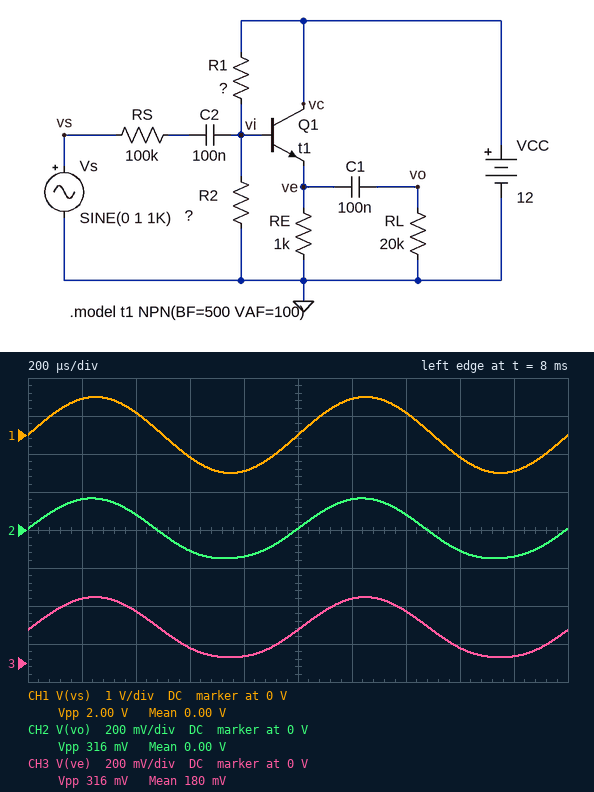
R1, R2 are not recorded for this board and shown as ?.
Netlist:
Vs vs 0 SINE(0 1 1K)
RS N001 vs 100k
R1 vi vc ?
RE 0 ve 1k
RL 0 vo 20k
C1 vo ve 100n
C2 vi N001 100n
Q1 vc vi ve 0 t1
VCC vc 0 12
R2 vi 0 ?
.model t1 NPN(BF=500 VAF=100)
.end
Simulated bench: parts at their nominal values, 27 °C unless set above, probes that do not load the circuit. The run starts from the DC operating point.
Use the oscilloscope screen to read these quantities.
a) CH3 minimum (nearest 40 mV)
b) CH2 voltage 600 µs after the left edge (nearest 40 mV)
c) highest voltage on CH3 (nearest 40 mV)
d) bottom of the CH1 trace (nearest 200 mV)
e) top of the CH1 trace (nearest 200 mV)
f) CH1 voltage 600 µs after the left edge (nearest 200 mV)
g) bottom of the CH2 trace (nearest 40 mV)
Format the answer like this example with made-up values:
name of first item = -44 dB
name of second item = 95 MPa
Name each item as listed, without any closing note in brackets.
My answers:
CH3 minimum = 40 mV
CH2 voltage 600 µs after the left edge = -120 mV
highest voltage on CH3 = 360 mV
bottom of the CH1 trace = -1.0 V
top of the CH1 trace = 1.0 V
CH1 voltage 600 µs after the left edge = -600 mV
bottom of the CH2 trace = -160 mV
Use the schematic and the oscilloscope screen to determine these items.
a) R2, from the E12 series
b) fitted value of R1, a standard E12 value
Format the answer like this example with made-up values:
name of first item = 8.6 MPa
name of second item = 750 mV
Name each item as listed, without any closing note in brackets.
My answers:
R2, from the E12 series = 27 kΩ
fitted value of R1, a standard E12 value = 330 kΩ
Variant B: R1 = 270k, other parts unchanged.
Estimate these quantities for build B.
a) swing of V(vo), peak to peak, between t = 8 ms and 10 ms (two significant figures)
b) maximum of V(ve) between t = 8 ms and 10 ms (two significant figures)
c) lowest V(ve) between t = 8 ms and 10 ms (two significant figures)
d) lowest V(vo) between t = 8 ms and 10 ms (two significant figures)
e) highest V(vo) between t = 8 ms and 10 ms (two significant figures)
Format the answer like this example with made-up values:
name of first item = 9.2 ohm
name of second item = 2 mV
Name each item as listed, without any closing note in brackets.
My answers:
swing of V(vo), peak to peak, between t = 8 ms and 10 ms = 350 mV
maximum of V(ve) between t = 8 ms and 10 ms = 510 mV
lowest V(ve) between t = 8 ms and 10 ms = 160 mV
lowest V(vo) between t = 8 ms and 10 ms = -170 mV
highest V(vo) between t = 8 ms and 10 ms = 180 mV
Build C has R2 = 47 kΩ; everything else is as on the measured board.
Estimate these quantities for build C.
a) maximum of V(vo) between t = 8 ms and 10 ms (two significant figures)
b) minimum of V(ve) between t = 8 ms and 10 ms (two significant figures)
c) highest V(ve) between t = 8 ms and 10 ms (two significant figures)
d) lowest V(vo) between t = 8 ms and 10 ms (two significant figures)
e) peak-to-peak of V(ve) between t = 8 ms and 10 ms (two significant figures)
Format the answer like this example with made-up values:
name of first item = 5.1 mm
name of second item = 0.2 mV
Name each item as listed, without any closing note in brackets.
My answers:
maximum of V(vo) between t = 8 ms and 10 ms = 270 mV
minimum of V(ve) between t = 8 ms and 10 ms = 420 mV
highest V(ve) between t = 8 ms and 10 ms = 950 mV
lowest V(vo) between t = 8 ms and 10 ms = -260 mV
peak-to-peak of V(ve) between t = 8 ms and 10 ms = 530 mV
